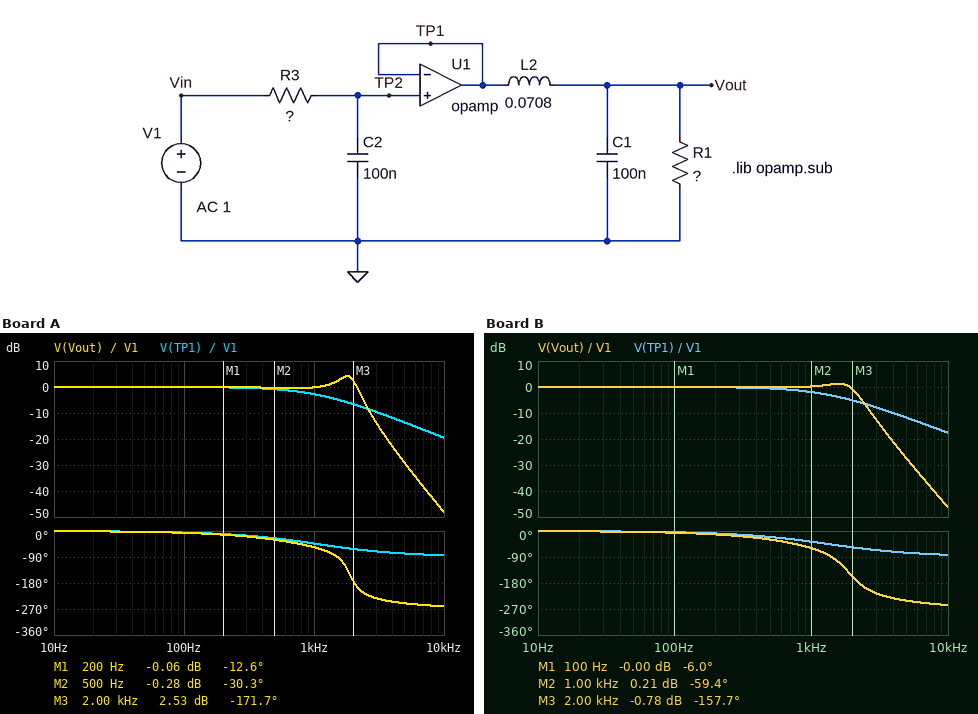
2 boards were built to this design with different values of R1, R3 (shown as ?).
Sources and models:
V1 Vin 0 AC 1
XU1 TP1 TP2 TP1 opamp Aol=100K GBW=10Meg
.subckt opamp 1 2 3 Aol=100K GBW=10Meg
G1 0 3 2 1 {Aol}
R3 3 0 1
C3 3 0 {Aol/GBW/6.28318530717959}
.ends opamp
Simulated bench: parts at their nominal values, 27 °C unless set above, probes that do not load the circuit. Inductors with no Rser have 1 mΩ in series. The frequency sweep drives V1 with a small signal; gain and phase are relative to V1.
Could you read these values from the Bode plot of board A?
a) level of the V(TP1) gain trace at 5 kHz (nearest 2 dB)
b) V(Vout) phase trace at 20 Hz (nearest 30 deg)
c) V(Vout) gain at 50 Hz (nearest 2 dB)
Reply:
-14 dB
0 deg
0 dB
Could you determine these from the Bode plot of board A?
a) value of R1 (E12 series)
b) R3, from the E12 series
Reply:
2.7 kΩ
1.5 kΩ
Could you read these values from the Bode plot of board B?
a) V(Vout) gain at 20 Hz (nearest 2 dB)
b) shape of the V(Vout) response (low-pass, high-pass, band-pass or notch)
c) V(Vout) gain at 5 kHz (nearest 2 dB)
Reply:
0 dB
low-pass
-28 dB
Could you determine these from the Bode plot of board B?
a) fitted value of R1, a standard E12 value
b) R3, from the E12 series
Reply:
1.5 kΩ
1.2 kΩ
